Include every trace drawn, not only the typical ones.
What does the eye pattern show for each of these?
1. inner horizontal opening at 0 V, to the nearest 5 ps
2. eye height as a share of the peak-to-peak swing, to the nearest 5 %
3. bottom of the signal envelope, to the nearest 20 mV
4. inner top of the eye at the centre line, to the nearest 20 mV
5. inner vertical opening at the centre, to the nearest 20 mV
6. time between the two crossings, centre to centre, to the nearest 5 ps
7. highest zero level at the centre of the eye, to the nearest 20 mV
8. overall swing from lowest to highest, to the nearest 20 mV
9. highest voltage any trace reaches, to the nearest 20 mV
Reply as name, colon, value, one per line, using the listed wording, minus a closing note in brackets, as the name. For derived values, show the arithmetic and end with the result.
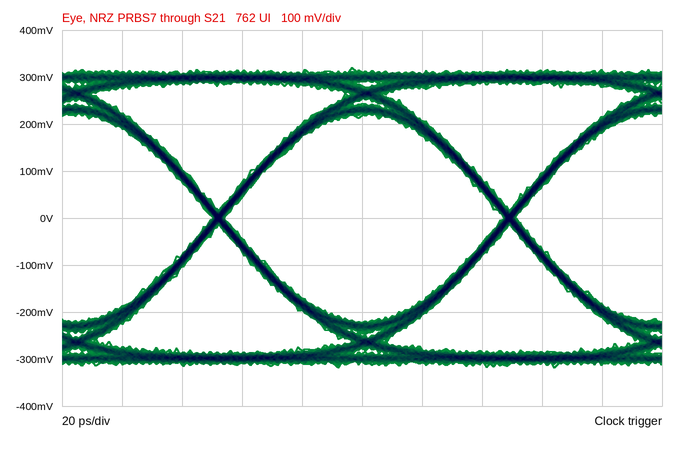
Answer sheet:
inner horizontal opening at 0 V, to the nearest 5 ps: 95 ps
eye height as a share of the peak-to-peak swing, to the nearest 5 %: 440 mV / 640 mV ≈ 68.8 %, so 70 % to the nearest 5 %
bottom of the signal envelope, to the nearest 20 mV: -320 mV
inner top of the eye at the centre line, to the nearest 20 mV: 220 mV
inner vertical opening at the centre, to the nearest 20 mV: 440 mV
time between the two crossings, centre to centre, to the nearest 5 ps: 95 ps
highest zero level at the centre of the eye, to the nearest 20 mV: -220 mV
overall swing from lowest to highest, to the nearest 20 mV: 640 mV
highest voltage any trace reaches, to the nearest 20 mV: 320 mV
